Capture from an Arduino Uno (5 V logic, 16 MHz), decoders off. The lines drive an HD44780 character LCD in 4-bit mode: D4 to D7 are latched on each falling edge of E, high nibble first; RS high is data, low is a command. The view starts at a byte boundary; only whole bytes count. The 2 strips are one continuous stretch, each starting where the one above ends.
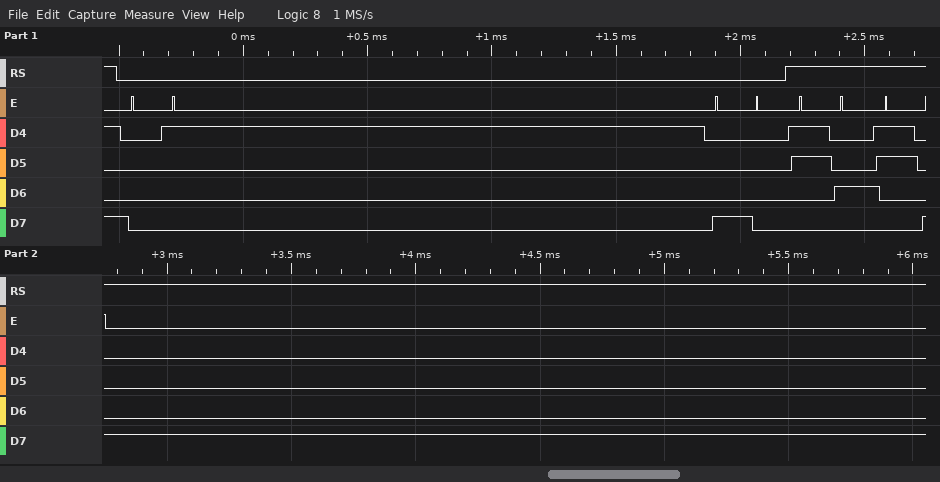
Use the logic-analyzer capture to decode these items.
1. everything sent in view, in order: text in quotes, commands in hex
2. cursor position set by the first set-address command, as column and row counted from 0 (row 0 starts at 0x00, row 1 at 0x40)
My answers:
0x01 0x80 "48"
column 0, row 0
